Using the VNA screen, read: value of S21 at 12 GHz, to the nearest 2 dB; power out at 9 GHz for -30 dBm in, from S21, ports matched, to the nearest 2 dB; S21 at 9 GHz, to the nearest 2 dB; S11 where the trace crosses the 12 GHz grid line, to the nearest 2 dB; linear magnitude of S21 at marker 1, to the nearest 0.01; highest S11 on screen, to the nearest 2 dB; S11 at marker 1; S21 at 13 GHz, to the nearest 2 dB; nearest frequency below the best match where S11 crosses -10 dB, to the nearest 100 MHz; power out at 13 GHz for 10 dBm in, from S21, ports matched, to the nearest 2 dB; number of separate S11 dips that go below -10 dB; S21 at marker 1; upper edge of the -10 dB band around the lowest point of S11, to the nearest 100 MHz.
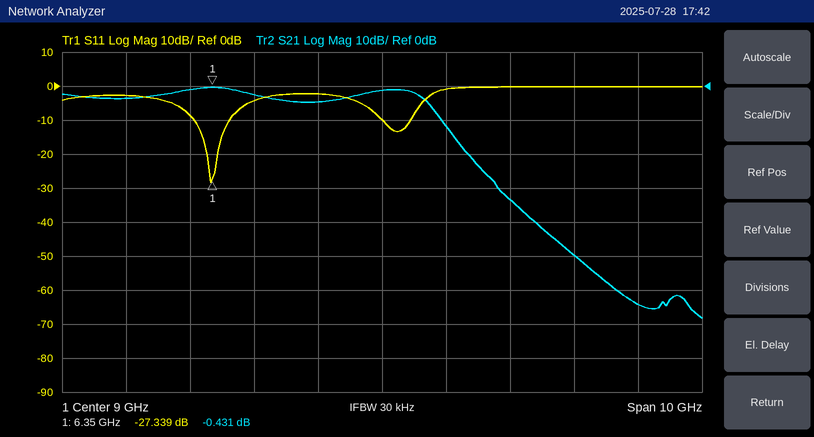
-50 dB
-32 dBm
-2 dB
0 dB
0.95
0 dB
-27.339 dB
-64 dB
6.1 GHz
-54 dBm
2
-0.431 dB
6.6 GHz
